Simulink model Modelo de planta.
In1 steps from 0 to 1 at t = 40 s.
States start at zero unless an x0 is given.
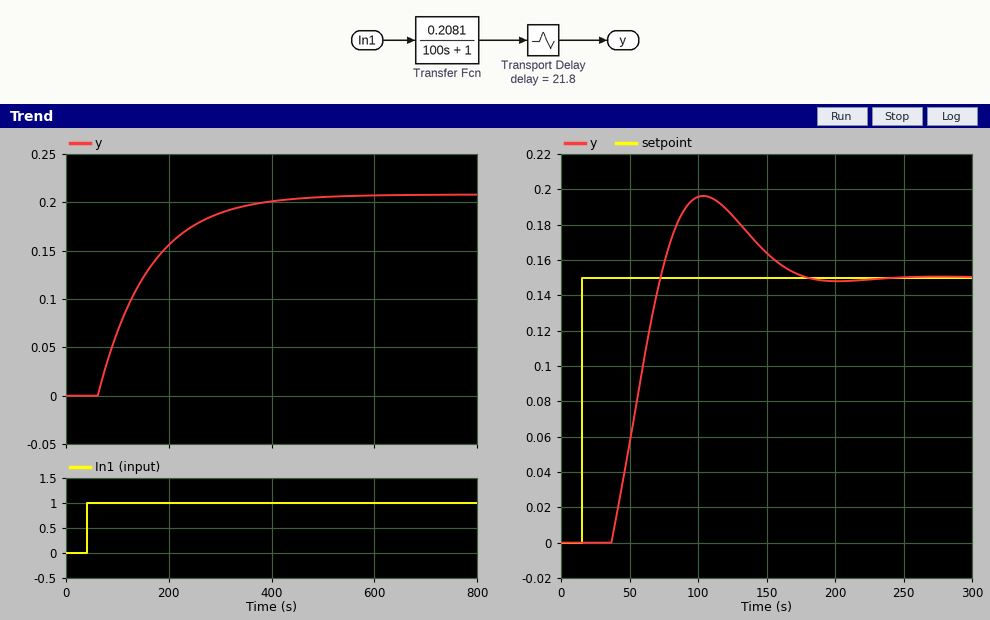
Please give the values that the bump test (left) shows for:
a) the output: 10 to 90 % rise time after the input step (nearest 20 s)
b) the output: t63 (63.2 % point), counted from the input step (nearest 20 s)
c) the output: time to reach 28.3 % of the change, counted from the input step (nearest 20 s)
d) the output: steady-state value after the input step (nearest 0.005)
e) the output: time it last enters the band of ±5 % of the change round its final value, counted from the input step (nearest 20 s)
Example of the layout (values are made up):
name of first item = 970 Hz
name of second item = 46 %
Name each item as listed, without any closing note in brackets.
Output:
the output: 10 to 90 % rise time after the input step = 220 s
the output: t63 (63.2 % point), counted from the input step = 120 s
the output: time to reach 28.3 % of the change, counted from the input step = 60 s
the output: steady-state value after the input step = 0.210
the output: time it last enters the band of ±5 % of the change round its final value, counted from the input step = 320 s
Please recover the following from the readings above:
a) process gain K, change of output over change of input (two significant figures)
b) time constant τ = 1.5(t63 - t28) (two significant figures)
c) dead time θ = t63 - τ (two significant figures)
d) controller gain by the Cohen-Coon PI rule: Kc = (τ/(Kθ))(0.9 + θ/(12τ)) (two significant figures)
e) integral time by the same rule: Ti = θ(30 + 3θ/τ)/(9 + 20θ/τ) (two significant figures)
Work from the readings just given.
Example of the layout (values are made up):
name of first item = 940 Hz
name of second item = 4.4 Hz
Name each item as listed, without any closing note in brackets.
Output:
process gain K, change of output over change of input = 0.21
time constant τ = 1.5(t63 - t28) = 90 s
dead time θ = t63 - τ = 30 s
controller gain by the Cohen-Coon PI rule: Kc = (τ/(Kθ))(0.9 + θ/(12τ)) = 13
integral time by the same rule: Ti = θ(30 + 3θ/τ)/(9 + 20θ/τ) = 59 s
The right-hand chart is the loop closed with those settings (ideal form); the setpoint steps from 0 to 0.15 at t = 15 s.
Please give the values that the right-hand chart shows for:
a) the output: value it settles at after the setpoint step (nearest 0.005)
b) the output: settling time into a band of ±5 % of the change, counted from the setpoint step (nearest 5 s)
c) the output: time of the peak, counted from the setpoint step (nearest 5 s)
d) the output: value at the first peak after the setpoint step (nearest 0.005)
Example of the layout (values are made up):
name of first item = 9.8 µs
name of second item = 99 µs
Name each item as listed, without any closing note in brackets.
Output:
the output: value it settles at after the setpoint step = 0.150
the output: settling time into a band of ±5 % of the change, counted from the setpoint step = 145 s
the output: time of the peak, counted from the setpoint step = 90 s
the output: value at the first peak after the setpoint step = 0.195
